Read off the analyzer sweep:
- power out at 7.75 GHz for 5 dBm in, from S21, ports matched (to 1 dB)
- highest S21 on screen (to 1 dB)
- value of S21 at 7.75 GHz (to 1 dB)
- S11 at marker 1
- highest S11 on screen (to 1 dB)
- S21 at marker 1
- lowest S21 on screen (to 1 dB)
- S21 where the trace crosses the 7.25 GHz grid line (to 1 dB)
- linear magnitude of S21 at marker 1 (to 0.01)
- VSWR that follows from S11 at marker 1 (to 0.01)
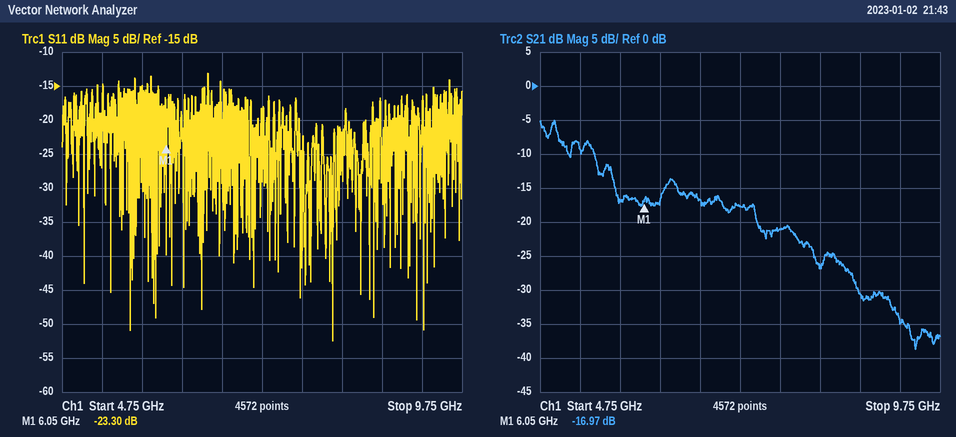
-16 dBm
-5 dB
-21 dB
-23.30 dB
-13 dB
-16.97 dB
-39 dB
-18 dB
0.14
1.15
